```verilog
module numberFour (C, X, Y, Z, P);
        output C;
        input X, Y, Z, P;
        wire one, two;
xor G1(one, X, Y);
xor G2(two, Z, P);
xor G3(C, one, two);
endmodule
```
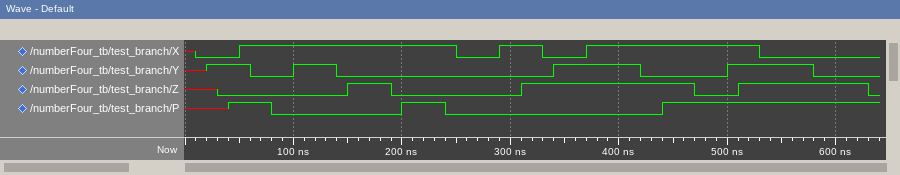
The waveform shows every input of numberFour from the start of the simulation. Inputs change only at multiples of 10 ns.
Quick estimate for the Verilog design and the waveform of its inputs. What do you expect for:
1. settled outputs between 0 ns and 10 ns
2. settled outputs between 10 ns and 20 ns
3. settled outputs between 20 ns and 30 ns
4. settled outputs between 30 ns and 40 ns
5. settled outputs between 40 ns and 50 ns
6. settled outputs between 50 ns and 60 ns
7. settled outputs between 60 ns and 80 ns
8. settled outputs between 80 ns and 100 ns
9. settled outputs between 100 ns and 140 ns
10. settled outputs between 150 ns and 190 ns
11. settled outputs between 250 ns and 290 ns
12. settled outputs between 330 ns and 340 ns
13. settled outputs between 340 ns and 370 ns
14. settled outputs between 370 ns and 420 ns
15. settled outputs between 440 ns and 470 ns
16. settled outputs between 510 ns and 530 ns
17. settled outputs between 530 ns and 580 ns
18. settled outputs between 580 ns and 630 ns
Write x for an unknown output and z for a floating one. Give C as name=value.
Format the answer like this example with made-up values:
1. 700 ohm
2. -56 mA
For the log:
1. C=x
2. C=x
3. C=x
4. C=x
5. C=0
6. C=1
7. C=0
8. C=1
9. C=0
10. C=0
11. C=0
12. C=1
13. C=0
14. C=1
15. C=1
16. C=0
17. C=1
18. C=0
